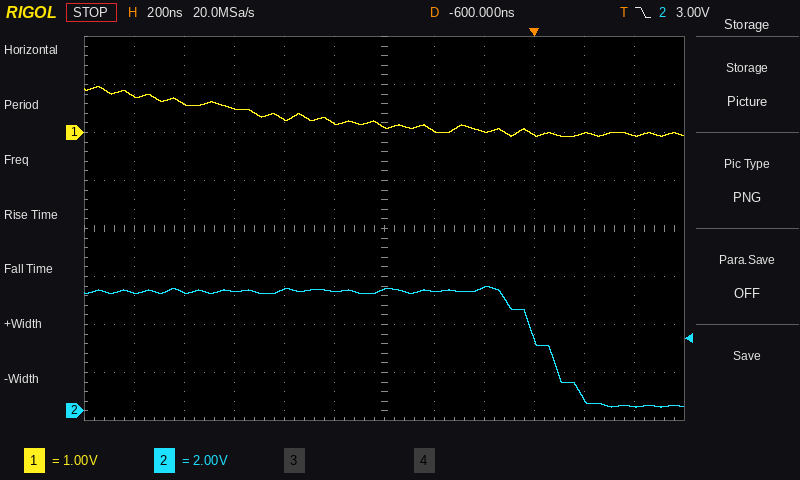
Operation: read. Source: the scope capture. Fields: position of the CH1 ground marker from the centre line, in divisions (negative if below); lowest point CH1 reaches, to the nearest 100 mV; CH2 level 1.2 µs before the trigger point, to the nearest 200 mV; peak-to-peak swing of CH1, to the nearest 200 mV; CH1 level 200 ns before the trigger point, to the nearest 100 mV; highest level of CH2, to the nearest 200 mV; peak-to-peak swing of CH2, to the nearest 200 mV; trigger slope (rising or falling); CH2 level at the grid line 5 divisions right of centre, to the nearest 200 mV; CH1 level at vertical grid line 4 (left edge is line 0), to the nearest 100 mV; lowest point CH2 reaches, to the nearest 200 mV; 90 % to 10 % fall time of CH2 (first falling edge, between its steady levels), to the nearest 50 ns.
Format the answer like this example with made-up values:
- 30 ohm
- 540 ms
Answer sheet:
- +2.0 div
- -100 mV
- 5.0 V
- 1.0 V
- 0.0 V
- 5.2 V
- 5.0 V
- falling
- 200 mV
- 300 mV
- 200 mV
- 300 ns
